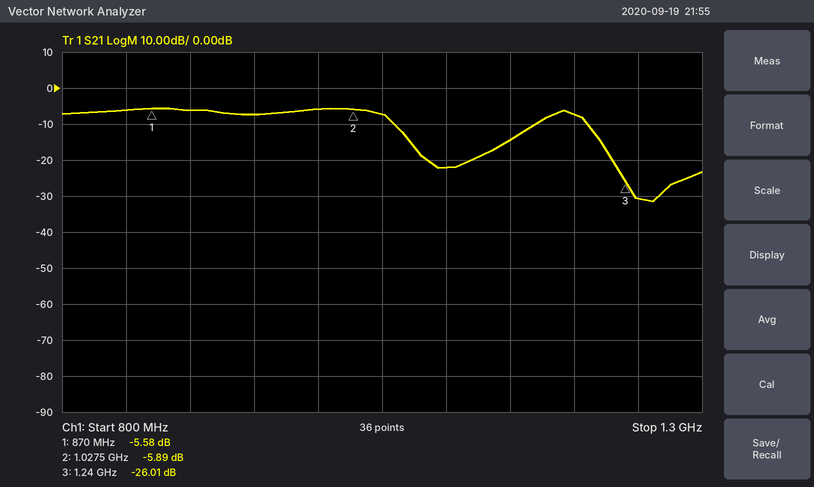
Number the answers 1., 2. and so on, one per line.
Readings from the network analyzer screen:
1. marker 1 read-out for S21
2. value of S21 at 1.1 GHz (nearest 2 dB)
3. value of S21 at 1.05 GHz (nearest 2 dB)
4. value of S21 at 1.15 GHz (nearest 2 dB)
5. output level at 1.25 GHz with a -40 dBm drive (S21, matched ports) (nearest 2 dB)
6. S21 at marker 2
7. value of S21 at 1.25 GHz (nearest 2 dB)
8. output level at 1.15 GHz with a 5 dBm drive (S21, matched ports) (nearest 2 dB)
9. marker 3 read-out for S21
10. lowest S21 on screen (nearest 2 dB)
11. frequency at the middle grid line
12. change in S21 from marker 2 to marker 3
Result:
1. -5.58 dB
2. -22 dB
3. -8 dB
4. -14 dB
5. -70 dBm
6. -5.89 dB
7. -30 dB
8. -10 dBm
9. -26.01 dB
10. -32 dB
11. 1.05 GHz
12. -20.12 dB
